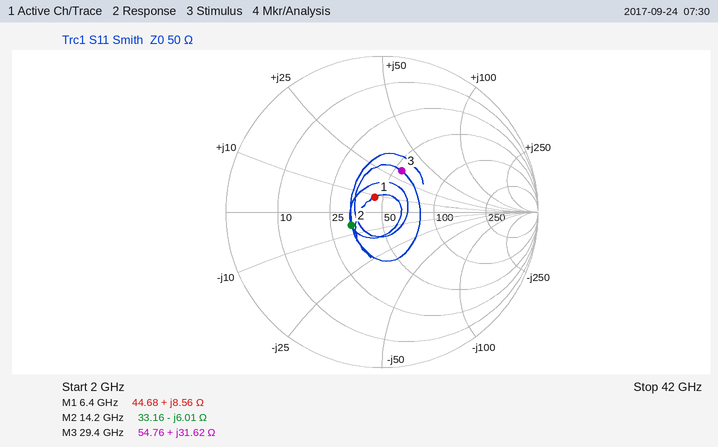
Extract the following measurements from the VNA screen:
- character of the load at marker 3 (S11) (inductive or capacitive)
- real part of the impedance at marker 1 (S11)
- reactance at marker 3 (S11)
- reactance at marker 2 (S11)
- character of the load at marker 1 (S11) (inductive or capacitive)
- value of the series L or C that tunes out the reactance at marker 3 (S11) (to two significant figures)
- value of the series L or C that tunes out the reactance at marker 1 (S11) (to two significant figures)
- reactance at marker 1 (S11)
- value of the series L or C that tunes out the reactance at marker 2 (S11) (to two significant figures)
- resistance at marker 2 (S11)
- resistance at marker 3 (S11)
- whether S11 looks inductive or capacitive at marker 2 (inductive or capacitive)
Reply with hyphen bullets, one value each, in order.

- inductive
- 44.68 Ω
- +31.62 Ω
- -6.01 Ω
- inductive
- 170 fF
- 2.9 pF
- +8.56 Ω
- 67 pH
- 33.16 Ω
- 54.76 Ω
- capacitive
